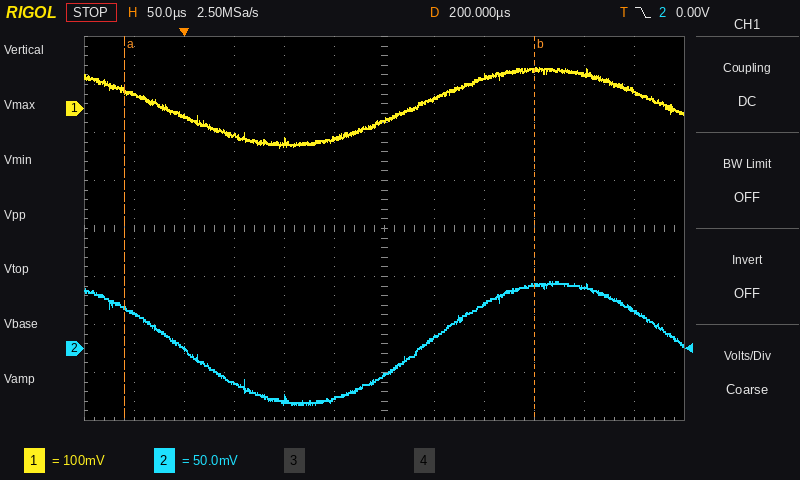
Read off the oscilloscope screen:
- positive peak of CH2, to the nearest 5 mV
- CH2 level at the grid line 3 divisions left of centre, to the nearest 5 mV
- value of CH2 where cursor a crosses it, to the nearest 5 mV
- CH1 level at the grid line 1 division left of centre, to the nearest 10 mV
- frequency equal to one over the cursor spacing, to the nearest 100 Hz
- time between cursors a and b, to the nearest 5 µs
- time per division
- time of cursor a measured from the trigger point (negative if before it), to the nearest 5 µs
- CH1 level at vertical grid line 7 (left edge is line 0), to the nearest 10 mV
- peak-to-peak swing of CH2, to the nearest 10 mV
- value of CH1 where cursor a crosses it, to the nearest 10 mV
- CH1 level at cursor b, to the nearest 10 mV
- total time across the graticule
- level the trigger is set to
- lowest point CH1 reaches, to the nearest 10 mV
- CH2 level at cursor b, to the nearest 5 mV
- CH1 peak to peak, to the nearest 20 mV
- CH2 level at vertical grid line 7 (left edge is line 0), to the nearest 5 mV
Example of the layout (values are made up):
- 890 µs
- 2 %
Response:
- 70 mV
- -35 mV
- 40 mV
- -60 mV
- 2.4 kHz
- 410 µs
- 50 µs
- -60 µs
- 20 mV
- 130 mV
- 40 mV
- 80 mV
- 600 µs
- 0.00 V
- -80 mV
- 65 mV
- 160 mV
- 10 mV
